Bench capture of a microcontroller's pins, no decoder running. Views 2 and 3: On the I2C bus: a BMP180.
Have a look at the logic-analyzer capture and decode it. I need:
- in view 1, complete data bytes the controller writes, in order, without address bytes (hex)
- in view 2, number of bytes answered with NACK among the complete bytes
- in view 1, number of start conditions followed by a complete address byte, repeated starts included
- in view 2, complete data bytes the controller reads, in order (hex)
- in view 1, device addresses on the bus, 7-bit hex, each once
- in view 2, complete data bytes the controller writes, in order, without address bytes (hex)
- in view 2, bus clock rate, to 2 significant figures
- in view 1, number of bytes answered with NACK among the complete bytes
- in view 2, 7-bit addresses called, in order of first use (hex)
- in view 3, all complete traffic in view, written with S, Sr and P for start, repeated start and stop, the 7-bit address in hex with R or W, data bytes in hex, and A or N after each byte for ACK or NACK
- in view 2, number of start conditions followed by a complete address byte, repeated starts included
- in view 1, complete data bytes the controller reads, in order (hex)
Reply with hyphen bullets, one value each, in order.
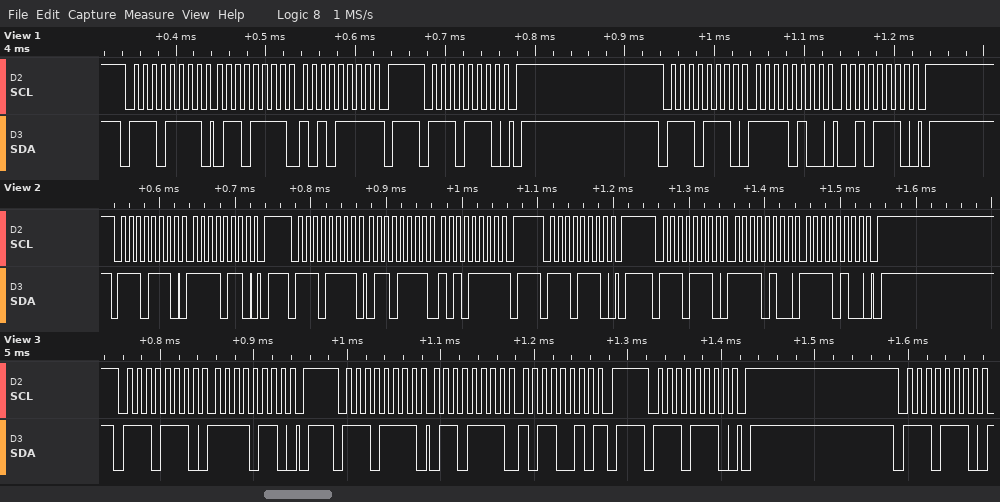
- F4 2E
- 1
- 3
- 6F AF
- 0x77
- F6 F4 F4
- 100 kHz
- 1
- 0x77
- S 77W A F6 A P S 77R A 6F A B2 N P S 77W A P S 77W A
- 4
- 6F AF
